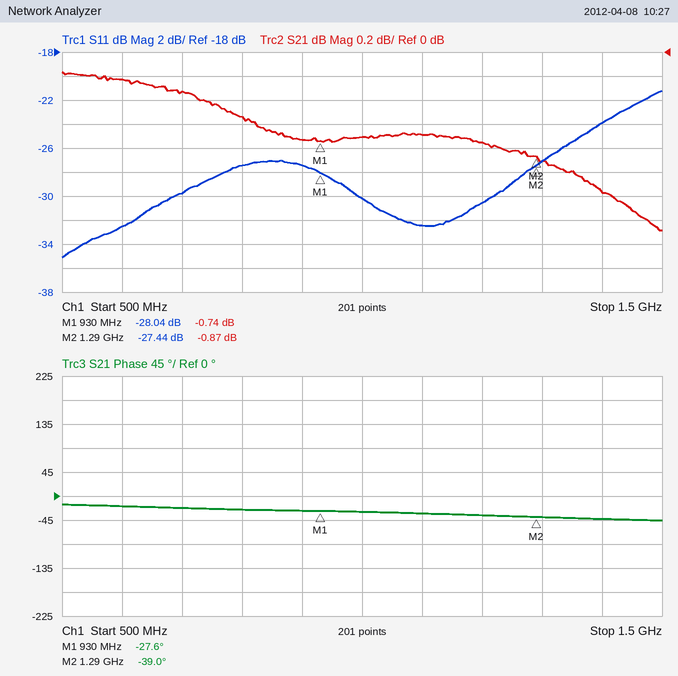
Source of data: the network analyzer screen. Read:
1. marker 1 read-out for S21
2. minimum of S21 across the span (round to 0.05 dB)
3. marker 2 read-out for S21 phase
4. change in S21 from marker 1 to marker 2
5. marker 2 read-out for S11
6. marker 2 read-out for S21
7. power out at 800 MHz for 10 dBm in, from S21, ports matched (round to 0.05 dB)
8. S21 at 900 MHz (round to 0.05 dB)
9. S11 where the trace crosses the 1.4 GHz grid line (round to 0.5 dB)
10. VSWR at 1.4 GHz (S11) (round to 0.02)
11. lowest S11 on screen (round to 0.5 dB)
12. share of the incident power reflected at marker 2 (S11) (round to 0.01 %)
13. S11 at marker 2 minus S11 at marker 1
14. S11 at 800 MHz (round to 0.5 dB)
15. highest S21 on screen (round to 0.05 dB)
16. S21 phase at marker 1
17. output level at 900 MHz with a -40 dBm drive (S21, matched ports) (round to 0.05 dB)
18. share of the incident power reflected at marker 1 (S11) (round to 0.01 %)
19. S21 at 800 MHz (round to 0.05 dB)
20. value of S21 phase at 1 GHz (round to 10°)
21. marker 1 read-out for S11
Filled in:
-0.74 dB
-1.50 dB
-39.0°
-0.13 dB
-27.44 dB
-0.87 dB
9.45 dBm
-0.75 dB
-24.0 dB
1.14
-35.0 dB
0.18 %
0.60 dB
-27.5 dB
-0.15 dB
-27.6°
-40.75 dBm
0.16 %
-0.55 dB
-30°
-28.04 dB
